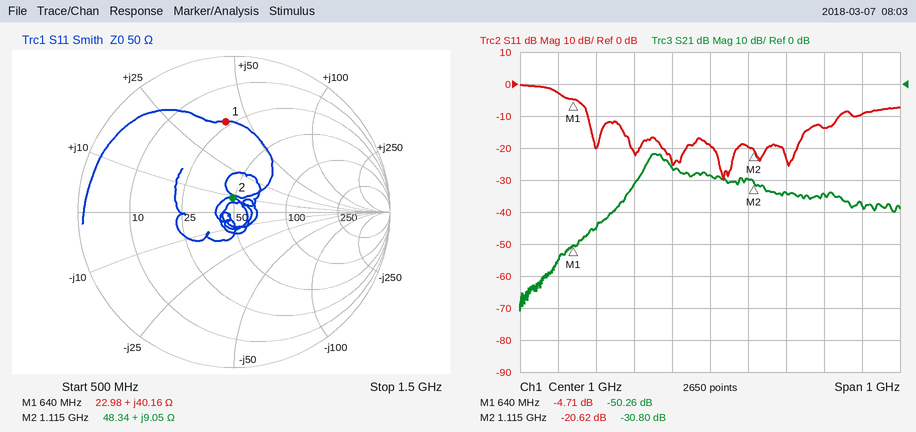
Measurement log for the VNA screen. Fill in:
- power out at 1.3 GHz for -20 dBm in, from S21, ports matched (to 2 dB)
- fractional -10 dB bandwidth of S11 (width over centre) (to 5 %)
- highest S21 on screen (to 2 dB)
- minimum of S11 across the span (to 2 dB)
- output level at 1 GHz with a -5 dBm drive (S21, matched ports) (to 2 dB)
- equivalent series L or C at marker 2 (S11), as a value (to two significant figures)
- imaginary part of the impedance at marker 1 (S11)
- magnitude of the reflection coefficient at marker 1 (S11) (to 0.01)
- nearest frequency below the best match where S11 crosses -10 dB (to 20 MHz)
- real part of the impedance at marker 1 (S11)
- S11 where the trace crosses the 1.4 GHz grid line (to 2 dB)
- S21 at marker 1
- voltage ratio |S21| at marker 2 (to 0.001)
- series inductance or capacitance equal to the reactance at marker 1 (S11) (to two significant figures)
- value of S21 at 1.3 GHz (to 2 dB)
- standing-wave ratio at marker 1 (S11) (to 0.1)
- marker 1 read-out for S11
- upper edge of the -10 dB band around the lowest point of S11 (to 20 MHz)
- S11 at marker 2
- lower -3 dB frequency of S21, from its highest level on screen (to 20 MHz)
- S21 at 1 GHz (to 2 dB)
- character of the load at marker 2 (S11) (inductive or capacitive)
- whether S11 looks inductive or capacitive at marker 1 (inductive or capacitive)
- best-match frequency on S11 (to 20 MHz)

-54 dBm
65 %
-22 dB
-30 dB
-34 dBm
1.3 nH
+40.16 Ω
0.58
680 MHz
22.98 Ω
-10 dB
-50.26 dB
0.029
10.0 nH
-34 dB
3.8
-4.71 dB
1.34 GHz
-20.62 dB
840 MHz
-28 dB
inductive
inductive
1.04 GHz
